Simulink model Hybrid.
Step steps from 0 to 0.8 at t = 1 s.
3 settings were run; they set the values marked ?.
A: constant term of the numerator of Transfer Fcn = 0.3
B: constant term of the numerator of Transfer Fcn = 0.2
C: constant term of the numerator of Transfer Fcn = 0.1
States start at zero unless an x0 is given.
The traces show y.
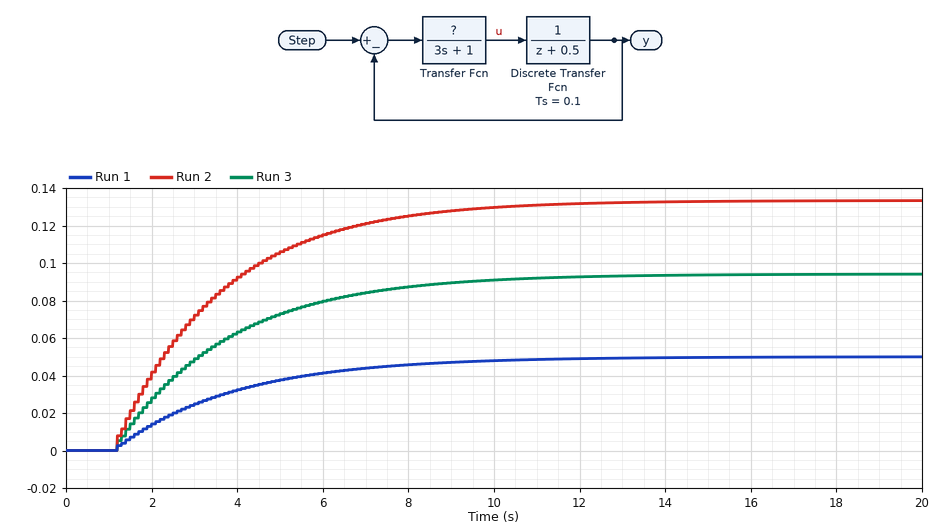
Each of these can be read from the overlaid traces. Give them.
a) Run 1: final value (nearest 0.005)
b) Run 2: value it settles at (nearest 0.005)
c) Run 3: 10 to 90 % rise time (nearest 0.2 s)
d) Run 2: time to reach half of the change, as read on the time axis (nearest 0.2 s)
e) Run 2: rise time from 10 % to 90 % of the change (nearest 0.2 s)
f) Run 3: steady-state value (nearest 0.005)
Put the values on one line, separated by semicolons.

0.050; 0.135; 5.8 s; 2.8 s; 5.4 s; 0.095
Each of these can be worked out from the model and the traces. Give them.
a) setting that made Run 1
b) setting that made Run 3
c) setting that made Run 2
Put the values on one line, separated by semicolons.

C; B; A
